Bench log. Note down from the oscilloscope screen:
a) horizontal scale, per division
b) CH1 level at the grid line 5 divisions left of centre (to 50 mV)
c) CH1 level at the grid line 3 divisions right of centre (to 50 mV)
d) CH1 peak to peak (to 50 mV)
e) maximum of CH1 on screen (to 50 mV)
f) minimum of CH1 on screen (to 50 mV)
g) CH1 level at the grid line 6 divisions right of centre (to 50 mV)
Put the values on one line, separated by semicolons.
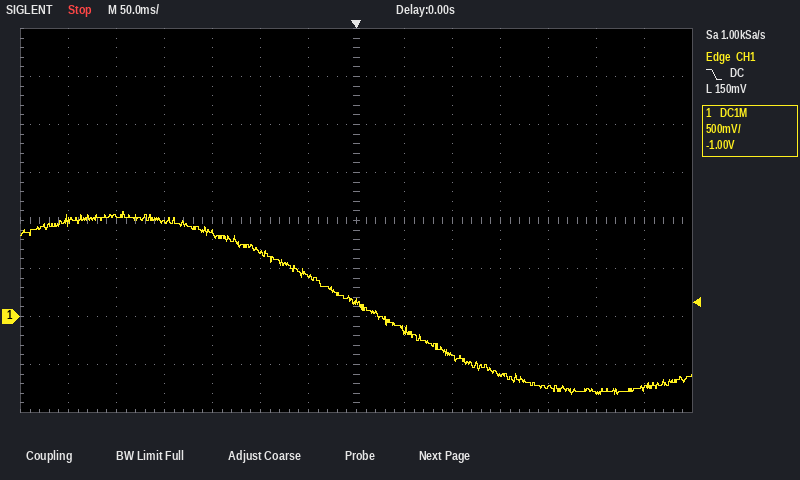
50 ms; 1.05 V; -600 mV; 1.90 V; 1.10 V; -800 mV; -750 mV
